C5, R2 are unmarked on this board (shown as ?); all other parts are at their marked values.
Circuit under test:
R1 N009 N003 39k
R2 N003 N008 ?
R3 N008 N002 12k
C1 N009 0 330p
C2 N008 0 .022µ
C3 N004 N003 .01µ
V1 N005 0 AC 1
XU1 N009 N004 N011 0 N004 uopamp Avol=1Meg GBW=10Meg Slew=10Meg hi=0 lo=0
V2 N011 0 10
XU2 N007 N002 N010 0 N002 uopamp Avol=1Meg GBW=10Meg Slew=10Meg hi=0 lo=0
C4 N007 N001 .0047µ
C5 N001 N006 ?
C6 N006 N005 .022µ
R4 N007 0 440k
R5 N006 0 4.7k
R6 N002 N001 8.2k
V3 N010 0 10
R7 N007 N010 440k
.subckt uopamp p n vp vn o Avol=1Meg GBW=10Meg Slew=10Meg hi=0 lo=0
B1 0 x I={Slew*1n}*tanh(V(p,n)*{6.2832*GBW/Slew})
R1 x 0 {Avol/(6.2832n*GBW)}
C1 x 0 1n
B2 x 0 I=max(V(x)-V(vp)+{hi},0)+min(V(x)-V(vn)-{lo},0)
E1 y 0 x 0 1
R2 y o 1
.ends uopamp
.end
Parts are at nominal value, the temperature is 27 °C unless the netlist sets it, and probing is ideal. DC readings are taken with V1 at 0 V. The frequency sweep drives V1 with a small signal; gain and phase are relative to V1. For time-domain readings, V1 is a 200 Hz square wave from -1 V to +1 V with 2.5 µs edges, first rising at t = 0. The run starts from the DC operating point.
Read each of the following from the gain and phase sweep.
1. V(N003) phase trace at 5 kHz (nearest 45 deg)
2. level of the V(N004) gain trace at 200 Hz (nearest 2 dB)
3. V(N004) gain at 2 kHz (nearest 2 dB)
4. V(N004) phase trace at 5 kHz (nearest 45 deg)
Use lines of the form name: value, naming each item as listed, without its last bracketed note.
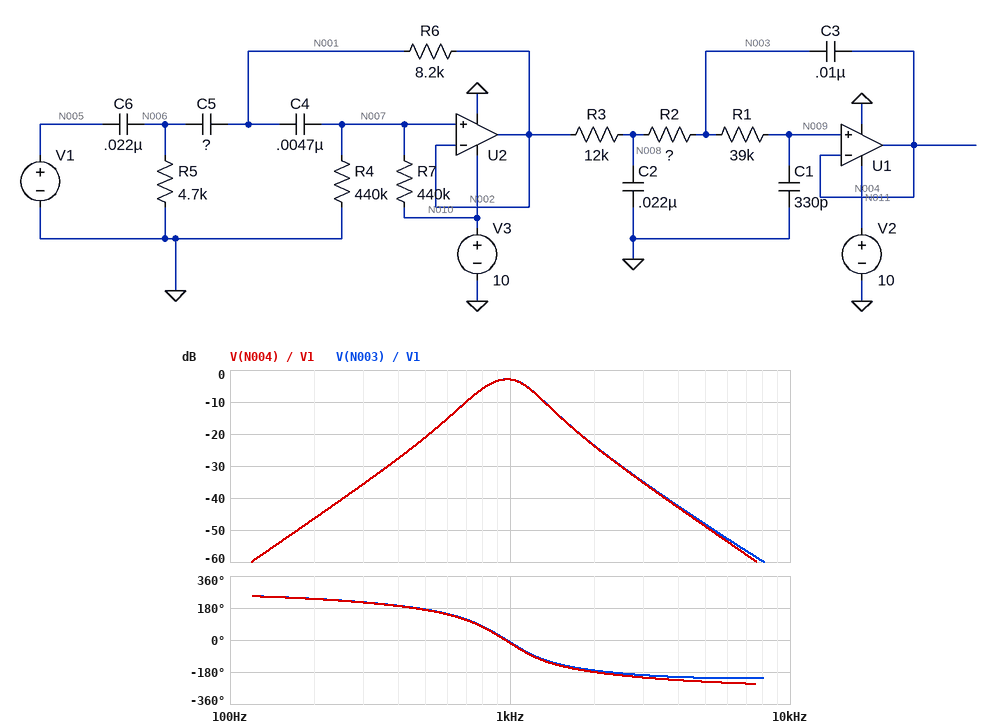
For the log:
V(N003) phase trace at 5 kHz: -225 deg
level of the V(N004) gain trace at 200 Hz: -46 dB
V(N004) gain at 2 kHz: -24 dB
V(N004) phase trace at 5 kHz: -225 deg
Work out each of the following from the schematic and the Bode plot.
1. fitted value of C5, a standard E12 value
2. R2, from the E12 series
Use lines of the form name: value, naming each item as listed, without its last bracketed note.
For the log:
fitted value of C5, a standard E12 value: 2.7 nF
R2, from the E12 series: 270 kΩ
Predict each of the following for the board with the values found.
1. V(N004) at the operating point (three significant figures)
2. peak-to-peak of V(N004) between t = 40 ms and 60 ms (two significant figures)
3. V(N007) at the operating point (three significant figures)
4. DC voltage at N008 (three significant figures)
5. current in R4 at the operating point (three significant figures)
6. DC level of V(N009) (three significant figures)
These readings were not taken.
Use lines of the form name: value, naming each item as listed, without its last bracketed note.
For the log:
V(N004) at the operating point: 5.00 V
peak-to-peak of V(N004) between t = 40 ms and 60 ms: 580 mV
V(N007) at the operating point: 5.00 V
DC voltage at N008: 5.00 V
current in R4 at the operating point: 11.4 µA
DC level of V(N009): 5.00 V
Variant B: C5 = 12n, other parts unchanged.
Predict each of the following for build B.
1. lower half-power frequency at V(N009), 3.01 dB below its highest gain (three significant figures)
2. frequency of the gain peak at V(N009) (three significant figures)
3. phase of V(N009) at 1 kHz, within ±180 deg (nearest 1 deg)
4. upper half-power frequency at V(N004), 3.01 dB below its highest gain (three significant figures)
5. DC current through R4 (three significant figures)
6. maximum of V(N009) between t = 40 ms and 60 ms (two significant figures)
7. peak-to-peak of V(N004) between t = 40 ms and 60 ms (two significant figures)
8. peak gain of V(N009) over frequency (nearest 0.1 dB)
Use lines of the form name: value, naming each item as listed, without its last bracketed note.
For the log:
lower half-power frequency at V(N009), 3.01 dB below its highest gain: 498 Hz
frequency of the gain peak at V(N009): 723 Hz
phase of V(N009) at 1 kHz, within ±180 deg: -100 deg
upper half-power frequency at V(N004), 3.01 dB below its highest gain: 951 Hz
DC current through R4: 11.4 µA
maximum of V(N009) between t = 40 ms and 60 ms: 5.4 V
peak-to-peak of V(N004) between t = 40 ms and 60 ms: 880 mV
peak gain of V(N009) over frequency: -2.4 dB
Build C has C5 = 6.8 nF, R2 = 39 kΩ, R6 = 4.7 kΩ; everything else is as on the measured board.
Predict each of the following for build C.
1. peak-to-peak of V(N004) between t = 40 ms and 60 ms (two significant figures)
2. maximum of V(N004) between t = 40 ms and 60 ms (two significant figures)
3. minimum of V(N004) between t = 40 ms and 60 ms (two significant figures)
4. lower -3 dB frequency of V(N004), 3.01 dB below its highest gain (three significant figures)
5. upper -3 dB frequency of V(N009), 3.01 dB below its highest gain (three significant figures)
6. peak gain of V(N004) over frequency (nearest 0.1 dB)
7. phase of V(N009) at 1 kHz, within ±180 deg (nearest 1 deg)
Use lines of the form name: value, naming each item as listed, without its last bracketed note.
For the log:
peak-to-peak of V(N004) between t = 40 ms and 60 ms: 1.1 V
maximum of V(N004) between t = 40 ms and 60 ms: 5.5 V
minimum of V(N004) between t = 40 ms and 60 ms: 4.5 V
lower -3 dB frequency of V(N004), 3.01 dB below its highest gain: 804 Hz
upper -3 dB frequency of V(N009), 3.01 dB below its highest gain: 2.23 kHz
peak gain of V(N004) over frequency: -1.7 dB
phase of V(N009) at 1 kHz, within ±180 deg: 49 deg
